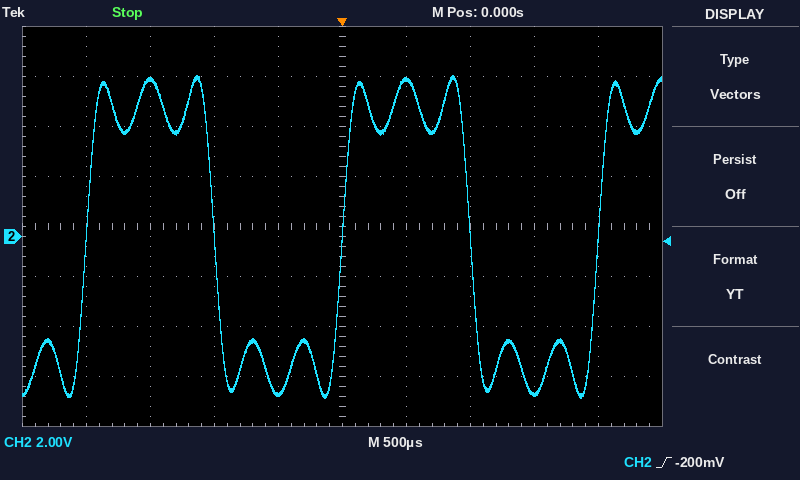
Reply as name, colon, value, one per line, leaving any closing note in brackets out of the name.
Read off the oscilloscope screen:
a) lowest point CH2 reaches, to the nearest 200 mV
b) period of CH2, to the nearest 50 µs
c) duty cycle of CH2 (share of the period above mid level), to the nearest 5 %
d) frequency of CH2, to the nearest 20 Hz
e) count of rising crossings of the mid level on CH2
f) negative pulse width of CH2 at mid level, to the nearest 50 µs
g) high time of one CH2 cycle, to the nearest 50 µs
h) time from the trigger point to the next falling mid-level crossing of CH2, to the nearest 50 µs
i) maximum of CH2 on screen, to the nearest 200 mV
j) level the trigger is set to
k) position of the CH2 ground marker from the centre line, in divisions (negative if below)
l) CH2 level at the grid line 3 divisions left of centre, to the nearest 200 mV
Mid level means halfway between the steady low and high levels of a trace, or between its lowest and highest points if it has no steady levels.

lowest point CH2 reaches, to the nearest 200 mV: -6.4 V
period of CH2, to the nearest 50 µs: 2.00 ms
duty cycle of CH2 (share of the period above mid level), to the nearest 5 %: 50 %
frequency of CH2, to the nearest 20 Hz: 500 Hz
count of rising crossings of the mid level on CH2: 3
negative pulse width of CH2 at mid level, to the nearest 50 µs: 1.00 ms
high time of one CH2 cycle, to the nearest 50 µs: 1.00 ms
time from the trigger point to the next falling mid-level crossing of CH2, to the nearest 50 µs: 1.00 ms
maximum of CH2 on screen, to the nearest 200 mV: 6.4 V
level the trigger is set to: -200 mV
position of the CH2 ground marker from the centre line, in divisions: -0.2 div
CH2 level at the grid line 3 divisions left of centre, to the nearest 200 mV: 6.2 V
